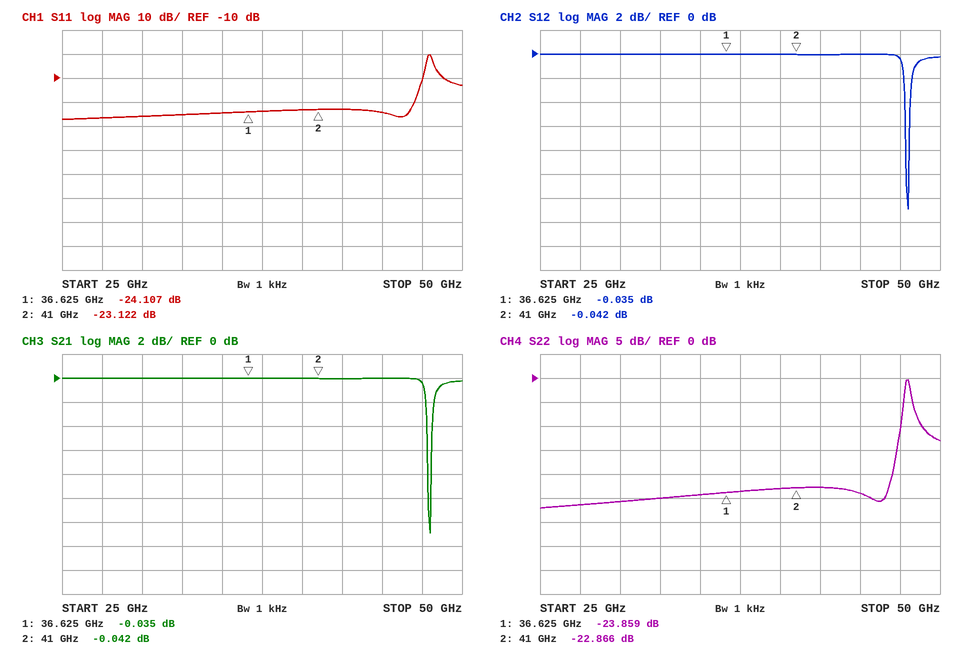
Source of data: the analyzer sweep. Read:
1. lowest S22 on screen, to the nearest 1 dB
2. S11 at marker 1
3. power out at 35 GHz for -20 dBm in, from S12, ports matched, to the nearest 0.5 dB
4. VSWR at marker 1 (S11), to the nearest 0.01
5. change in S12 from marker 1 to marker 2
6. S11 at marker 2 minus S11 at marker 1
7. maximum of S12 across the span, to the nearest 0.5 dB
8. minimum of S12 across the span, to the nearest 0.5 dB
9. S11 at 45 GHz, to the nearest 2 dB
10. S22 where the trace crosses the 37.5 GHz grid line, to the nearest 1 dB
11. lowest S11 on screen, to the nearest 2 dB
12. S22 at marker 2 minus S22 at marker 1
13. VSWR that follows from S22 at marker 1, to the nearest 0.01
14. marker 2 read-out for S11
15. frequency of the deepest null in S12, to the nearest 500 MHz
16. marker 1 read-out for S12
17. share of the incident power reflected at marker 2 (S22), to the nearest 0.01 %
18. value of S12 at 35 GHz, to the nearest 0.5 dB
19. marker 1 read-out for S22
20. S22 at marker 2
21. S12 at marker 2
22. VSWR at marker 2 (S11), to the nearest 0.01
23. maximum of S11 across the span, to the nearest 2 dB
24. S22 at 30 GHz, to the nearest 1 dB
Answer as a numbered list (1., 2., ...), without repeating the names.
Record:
1. -27 dB
2. -24.107 dB
3. -20.0 dBm
4. 1.13
5. -0.007 dB
6. 0.985 dB
7. 0.0 dB
8. -13.0 dB
9. -24 dB
10. -24 dB
11. -28 dB
12. 0.993 dB
13. 1.14
14. -23.122 dB
15. 48.0 GHz
16. -0.035 dB
17. 0.52 %
18. 0.0 dB
19. -23.859 dB
20. -22.866 dB
21. -0.042 dB
22. 1.15
23. 0 dB
24. -26 dB
